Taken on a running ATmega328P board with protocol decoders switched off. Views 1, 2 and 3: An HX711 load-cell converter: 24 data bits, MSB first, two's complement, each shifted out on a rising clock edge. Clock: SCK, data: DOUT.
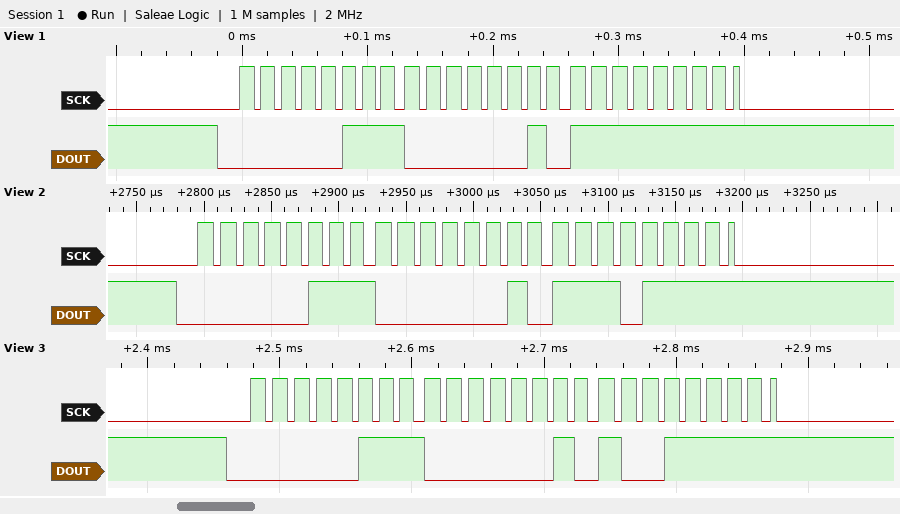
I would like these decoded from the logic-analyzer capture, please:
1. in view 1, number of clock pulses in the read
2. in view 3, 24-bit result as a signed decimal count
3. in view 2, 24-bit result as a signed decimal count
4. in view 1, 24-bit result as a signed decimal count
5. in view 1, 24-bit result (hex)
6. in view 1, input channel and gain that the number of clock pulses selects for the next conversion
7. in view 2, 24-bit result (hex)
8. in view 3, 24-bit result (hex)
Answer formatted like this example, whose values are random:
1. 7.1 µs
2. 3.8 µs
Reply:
1. 25
2. 459423
3. 459503
4. 459519
5. 0x0702FF
6. channel A, gain 128
7. 0x0702EF
8. 0x07029F
